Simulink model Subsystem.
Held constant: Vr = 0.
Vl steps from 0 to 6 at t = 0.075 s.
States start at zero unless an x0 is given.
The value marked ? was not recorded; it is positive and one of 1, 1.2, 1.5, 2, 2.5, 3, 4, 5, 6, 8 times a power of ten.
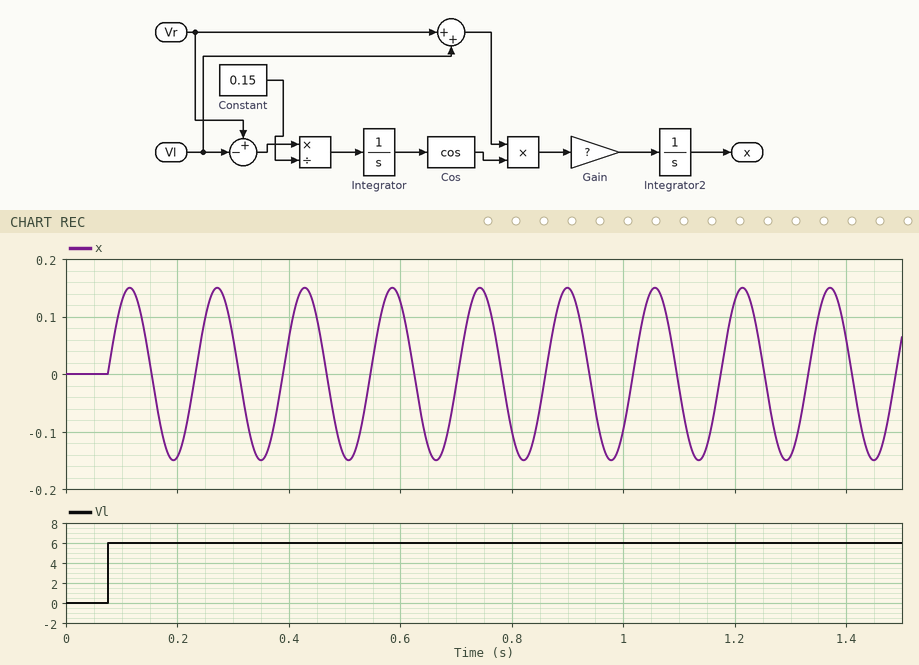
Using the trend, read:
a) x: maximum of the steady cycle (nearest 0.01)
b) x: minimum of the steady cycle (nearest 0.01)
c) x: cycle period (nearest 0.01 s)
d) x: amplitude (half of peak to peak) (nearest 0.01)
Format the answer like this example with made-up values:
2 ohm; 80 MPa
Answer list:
0.15; -0.15; 0.16 s; 0.15
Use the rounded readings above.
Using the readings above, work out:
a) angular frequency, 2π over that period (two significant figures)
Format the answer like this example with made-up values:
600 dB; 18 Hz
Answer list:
39 rad/s
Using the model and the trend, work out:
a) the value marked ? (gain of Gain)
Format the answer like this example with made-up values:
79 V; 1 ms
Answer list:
1
